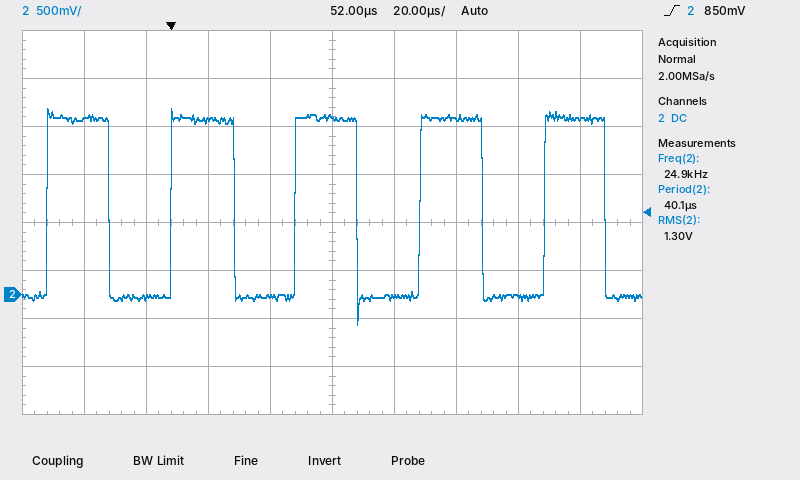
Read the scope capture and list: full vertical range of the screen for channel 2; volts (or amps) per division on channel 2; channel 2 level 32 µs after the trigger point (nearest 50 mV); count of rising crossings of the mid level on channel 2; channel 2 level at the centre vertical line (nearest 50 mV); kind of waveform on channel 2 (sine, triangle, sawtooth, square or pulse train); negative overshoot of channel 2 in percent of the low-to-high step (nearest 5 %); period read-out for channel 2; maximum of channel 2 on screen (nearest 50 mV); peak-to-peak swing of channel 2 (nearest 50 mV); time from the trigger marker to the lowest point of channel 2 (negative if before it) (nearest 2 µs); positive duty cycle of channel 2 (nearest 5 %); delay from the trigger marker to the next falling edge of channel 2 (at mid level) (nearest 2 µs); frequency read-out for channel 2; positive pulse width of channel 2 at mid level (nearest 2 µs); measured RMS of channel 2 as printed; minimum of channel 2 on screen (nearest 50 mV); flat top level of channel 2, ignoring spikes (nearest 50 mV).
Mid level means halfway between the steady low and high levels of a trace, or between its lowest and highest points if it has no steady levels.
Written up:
4 V
500 mV
0 mV
5
1.85 V
square
15 %
40.1 µs
1.95 V
2.25 V
+60 µs
50 %
20 µs
24.9 kHz
20 µs
1.30 V
-300 mV
1.85 V
